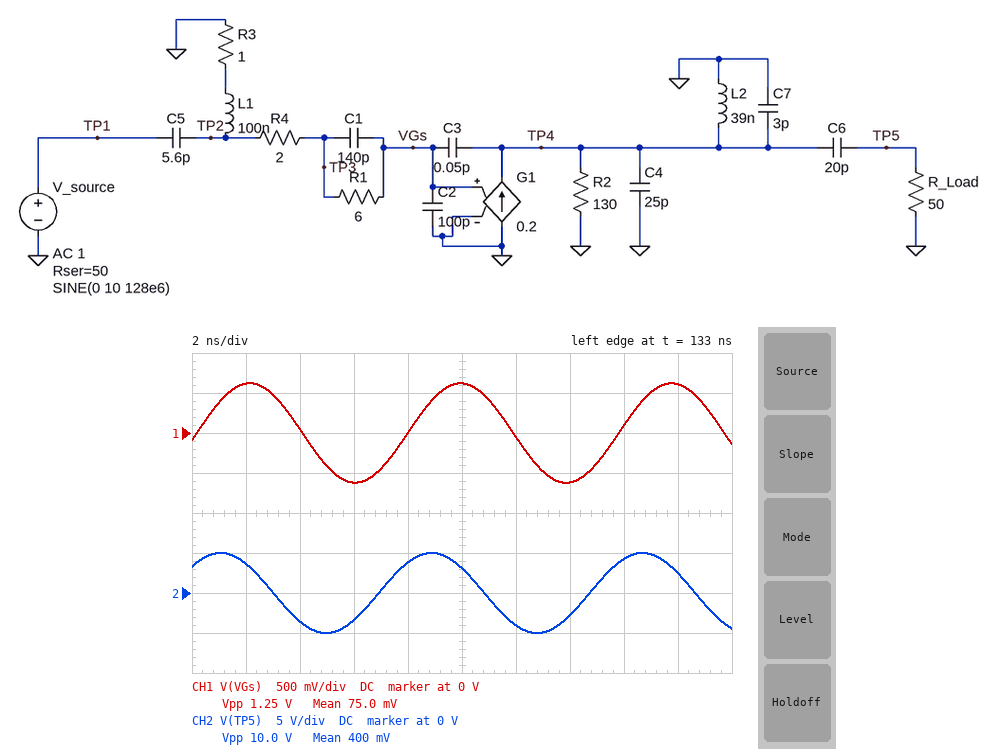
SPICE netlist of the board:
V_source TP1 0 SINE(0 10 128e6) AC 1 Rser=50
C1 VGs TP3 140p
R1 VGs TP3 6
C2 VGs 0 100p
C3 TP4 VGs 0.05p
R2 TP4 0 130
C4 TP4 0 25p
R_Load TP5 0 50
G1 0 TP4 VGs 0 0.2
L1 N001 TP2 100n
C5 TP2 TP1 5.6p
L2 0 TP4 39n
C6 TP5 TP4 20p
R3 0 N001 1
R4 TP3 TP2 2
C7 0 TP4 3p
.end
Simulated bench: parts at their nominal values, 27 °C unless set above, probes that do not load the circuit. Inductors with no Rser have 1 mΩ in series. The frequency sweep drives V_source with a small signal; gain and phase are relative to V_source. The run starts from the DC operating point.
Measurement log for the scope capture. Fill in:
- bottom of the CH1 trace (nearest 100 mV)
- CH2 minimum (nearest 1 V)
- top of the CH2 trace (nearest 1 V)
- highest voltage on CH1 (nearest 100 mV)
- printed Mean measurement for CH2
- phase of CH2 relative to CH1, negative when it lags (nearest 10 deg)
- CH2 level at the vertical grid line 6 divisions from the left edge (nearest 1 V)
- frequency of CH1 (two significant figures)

-600 mV
-5 V
5 V
600 mV
400 mV
50 deg
-4 V
130 MHz
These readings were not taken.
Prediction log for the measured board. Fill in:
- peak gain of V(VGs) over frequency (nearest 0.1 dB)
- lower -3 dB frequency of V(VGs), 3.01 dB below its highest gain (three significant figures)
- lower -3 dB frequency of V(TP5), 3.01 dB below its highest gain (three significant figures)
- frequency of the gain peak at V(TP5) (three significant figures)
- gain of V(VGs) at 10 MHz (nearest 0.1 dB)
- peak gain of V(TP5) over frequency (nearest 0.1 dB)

-13.6 dB
45.2 MHz
96.4 MHz
123 MHz
-52.7 dB
-5.9 dB
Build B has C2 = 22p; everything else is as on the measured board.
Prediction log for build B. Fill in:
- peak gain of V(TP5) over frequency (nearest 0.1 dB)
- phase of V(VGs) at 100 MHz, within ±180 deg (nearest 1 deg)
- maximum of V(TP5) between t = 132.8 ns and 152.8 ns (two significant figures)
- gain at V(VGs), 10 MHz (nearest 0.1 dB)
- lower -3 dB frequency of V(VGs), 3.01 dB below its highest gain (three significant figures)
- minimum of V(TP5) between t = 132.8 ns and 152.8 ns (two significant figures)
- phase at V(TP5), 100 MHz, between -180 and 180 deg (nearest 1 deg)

18.0 dB
61 deg
39 V
-52.9 dB
91.8 MHz
-39 V
166 deg
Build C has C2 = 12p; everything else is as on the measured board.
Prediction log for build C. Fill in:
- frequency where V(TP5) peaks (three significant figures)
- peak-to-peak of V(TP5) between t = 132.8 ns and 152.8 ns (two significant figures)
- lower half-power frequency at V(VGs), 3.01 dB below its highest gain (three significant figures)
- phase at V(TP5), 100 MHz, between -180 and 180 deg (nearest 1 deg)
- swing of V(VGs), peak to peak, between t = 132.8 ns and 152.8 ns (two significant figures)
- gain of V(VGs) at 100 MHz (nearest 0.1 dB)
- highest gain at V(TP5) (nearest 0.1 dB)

125 MHz
390 V
117 MHz
-103 deg
48 V
-4.2 dB
26.5 dB
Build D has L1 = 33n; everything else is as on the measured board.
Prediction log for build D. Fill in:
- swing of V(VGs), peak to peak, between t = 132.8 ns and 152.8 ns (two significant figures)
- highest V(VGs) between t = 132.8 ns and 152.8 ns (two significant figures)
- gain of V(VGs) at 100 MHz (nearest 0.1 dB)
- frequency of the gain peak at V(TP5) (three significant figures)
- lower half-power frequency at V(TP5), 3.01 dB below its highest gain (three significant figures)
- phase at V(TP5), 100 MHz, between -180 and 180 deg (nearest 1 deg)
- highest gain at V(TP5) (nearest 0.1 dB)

2.0 V
980 mV
-17.3 dB
115 MHz
93.0 MHz
156 deg
-1.3 dB
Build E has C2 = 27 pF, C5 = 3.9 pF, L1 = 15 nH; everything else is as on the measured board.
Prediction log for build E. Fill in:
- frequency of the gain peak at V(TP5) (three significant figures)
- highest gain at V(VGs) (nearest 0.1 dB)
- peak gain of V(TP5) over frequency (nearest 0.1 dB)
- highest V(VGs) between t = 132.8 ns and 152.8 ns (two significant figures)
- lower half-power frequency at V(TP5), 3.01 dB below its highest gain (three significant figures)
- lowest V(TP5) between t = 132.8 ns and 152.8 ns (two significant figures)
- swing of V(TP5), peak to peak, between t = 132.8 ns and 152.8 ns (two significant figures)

247 MHz
-4.9 dB
7.0 dB
480 mV
221 MHz
-3.9 V
7.8 V
